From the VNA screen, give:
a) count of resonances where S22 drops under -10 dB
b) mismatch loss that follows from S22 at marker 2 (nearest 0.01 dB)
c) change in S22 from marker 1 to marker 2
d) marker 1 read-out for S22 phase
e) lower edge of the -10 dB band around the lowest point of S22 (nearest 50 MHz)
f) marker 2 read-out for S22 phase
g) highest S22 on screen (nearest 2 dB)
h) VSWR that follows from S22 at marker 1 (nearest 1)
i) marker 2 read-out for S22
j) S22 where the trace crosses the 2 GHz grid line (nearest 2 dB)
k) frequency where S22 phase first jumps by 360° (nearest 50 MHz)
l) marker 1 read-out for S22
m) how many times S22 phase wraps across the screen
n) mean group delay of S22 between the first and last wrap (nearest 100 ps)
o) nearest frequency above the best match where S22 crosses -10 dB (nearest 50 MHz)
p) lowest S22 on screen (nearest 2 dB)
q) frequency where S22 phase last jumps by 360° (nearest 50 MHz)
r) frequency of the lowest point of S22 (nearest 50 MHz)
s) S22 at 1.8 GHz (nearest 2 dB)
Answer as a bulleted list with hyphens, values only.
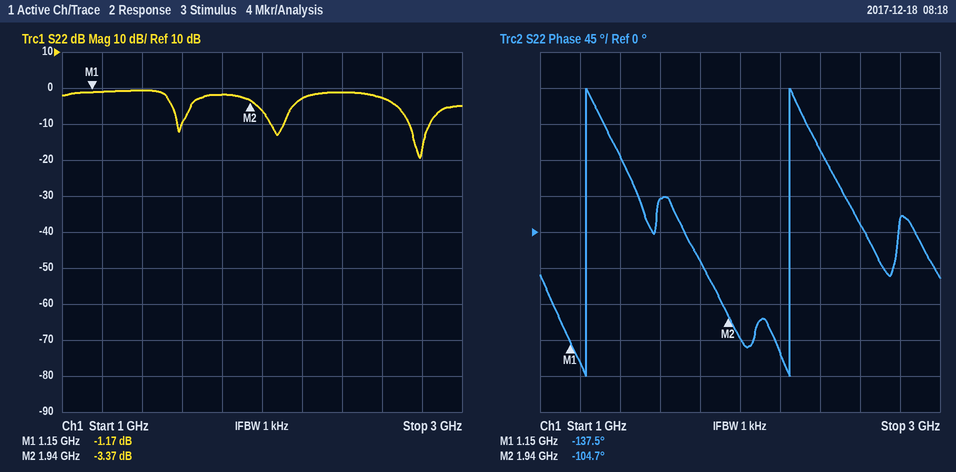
- 3
- 2.68 dB
- -2.20 dB
- -137.5°
- 2.75 GHz
- -104.7°
- 0 dB
- 15
- -3.37 dB
- -6 dB
- 1.25 GHz
- -1.17 dB
- 2
- 1.0 ns
- 2.85 GHz
- -20 dB
- 2.25 GHz
- 2.80 GHz
- -2 dB
